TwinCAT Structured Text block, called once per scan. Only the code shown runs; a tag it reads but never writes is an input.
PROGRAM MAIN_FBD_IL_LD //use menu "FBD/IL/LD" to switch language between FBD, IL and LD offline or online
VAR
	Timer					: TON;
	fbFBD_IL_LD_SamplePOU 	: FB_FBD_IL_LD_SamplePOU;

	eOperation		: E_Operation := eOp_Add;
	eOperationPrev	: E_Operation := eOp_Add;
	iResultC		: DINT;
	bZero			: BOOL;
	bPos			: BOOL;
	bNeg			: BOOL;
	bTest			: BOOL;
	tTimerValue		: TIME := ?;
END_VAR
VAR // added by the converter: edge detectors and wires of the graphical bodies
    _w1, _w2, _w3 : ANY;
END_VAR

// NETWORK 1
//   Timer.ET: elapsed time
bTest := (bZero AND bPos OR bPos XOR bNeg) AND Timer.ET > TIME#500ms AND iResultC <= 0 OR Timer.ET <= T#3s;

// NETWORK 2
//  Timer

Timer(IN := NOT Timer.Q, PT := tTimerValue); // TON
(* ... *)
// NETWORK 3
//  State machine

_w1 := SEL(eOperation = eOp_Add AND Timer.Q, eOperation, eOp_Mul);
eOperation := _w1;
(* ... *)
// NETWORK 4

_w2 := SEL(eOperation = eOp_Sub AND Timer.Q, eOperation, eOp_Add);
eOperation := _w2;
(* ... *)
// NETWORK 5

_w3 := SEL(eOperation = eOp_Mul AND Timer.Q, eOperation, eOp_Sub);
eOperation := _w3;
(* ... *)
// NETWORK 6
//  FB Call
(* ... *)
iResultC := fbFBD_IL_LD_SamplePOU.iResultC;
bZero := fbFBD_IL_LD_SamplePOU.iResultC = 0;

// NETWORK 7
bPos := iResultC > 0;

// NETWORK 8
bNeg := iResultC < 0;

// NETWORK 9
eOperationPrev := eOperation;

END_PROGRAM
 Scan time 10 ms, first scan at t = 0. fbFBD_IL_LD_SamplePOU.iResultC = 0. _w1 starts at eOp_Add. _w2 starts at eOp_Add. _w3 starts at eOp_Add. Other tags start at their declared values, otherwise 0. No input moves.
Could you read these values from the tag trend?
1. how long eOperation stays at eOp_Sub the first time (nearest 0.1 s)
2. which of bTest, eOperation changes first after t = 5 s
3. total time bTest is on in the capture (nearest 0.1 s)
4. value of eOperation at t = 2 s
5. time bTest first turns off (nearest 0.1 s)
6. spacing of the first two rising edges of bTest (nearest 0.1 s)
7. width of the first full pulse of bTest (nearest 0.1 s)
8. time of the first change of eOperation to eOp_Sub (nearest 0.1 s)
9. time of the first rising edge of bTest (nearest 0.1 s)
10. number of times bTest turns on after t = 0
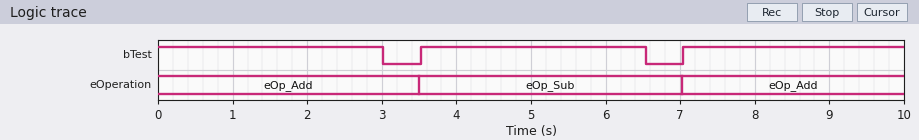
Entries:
3.5 s
bTest
9.0 s
eOp_Add
3.0 s
3.5 s
3.0 s
3.5 s
3.5 s
2
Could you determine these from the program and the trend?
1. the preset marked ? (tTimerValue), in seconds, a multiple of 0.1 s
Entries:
3.5 s
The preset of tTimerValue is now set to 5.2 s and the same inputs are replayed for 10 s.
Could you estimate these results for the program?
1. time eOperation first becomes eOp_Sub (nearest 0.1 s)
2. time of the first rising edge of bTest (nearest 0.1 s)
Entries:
5.2 s
5.2 s
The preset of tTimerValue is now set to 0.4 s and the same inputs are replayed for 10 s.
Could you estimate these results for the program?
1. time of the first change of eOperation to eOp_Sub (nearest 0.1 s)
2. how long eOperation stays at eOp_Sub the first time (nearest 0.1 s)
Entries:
0.4 s
0.4 s
